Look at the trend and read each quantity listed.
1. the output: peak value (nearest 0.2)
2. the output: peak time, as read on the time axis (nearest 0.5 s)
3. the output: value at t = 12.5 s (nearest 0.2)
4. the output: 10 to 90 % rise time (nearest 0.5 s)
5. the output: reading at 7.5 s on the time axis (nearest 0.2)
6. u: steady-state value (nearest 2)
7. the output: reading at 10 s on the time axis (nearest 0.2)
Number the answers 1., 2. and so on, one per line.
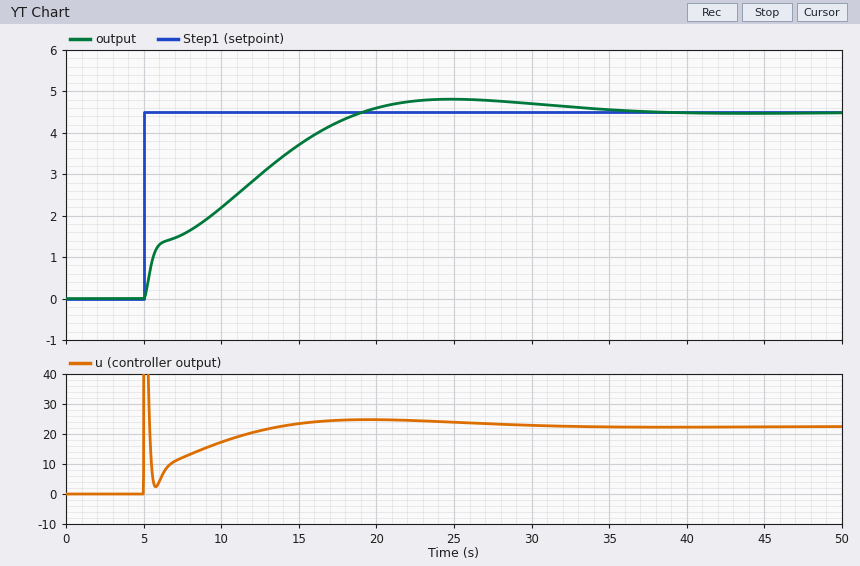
1. 4.8
2. 25.0 s
3. 3.0
4. 11.0 s
5. 1.6
6. 22
7. 2.2
